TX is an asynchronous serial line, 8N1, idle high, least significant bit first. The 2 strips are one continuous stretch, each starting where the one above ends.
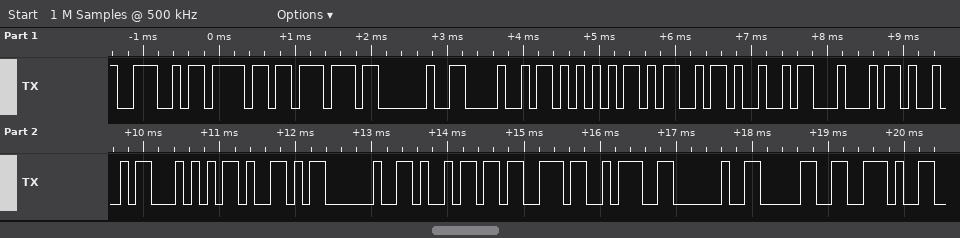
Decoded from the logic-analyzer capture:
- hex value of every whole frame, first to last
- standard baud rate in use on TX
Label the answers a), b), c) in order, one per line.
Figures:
a) 0x4E 0x6F 0x77 0x20 0x48 0x55 0x4D 0x49 0x44 0x49 0x54 0x59 0x20 0x69 0x73 0x3A 0x20 0x30 0x2E
b) 9600 baud
